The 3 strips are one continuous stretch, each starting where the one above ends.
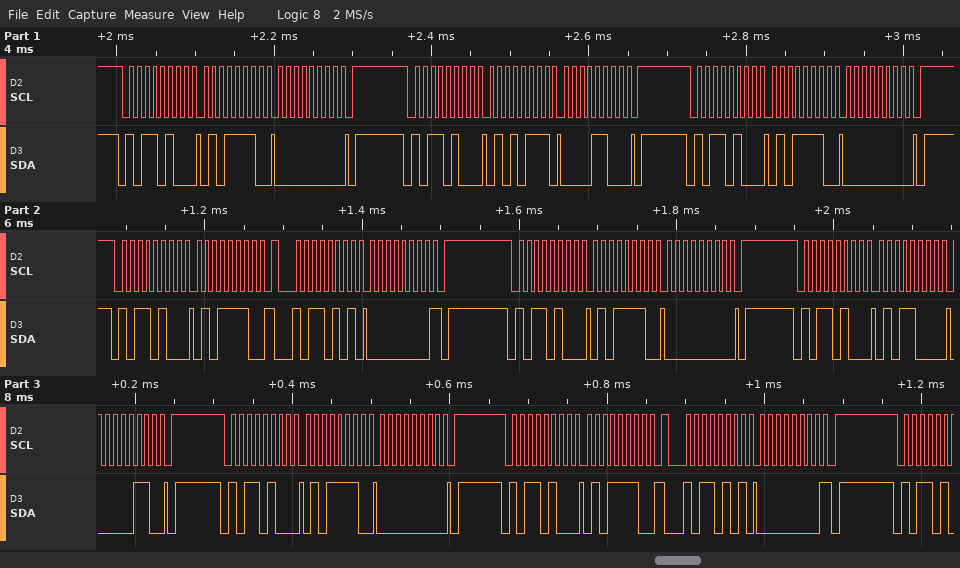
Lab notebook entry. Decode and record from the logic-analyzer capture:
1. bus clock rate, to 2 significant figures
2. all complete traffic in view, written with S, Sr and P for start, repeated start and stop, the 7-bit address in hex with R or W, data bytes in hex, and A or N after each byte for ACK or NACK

100 kHz
S 5AW A 5E A 00 A P S 5AW A 57 A 0C A P S 5AW A 5E A 00 A P S 5AW A 5E A Sr 5AR A 00 N P S 5AW A 5E A 00 A P S 5AW A 58 A 06 A P S 5AW A 5E A 00 A P S 5AW A 5E A Sr 5AR A 00 N P
